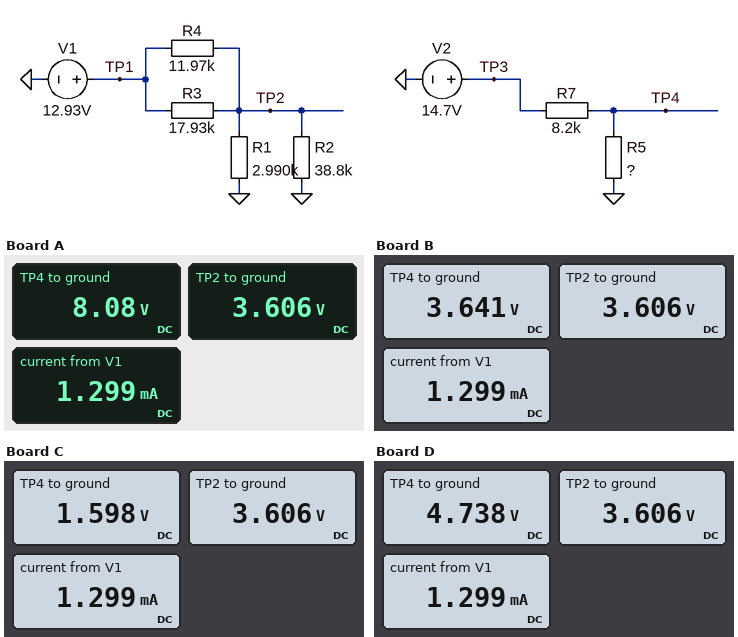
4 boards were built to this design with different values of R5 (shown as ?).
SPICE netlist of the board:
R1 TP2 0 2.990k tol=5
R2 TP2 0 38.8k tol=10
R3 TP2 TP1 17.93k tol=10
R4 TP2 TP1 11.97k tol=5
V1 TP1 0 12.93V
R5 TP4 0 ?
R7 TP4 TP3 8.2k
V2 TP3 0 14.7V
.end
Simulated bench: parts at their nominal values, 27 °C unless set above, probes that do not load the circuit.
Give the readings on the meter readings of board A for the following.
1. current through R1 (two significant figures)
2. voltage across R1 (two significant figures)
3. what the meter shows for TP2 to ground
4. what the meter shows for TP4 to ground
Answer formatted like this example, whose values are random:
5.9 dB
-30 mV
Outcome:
1.2 mA
3.6 V
3.606 V
8.08 V
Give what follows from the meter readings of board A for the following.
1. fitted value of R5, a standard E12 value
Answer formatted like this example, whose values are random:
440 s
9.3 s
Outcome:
10 kΩ
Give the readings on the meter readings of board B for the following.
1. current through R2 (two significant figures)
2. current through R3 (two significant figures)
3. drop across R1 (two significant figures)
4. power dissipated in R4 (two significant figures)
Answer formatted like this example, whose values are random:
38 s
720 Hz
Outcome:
93 µA
520 µA
3.6 V
7.3 mW
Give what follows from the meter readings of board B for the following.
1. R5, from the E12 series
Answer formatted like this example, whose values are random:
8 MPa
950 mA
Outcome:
2.7 kΩ
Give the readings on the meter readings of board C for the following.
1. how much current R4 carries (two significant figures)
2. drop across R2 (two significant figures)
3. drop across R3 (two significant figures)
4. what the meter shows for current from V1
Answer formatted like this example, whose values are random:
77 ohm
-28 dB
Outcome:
780 µA
3.6 V
9.3 V
1.299 mA
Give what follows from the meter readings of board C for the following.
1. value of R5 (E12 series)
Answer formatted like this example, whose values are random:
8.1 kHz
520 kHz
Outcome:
1 kΩ
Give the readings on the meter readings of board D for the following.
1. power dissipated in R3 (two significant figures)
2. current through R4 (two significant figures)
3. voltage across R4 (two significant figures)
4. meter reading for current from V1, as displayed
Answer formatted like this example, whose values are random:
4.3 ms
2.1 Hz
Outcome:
4.8 mW
780 µA
9.3 V
1.299 mA
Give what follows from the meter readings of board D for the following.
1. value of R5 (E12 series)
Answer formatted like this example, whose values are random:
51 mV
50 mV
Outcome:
3.9 kΩ
